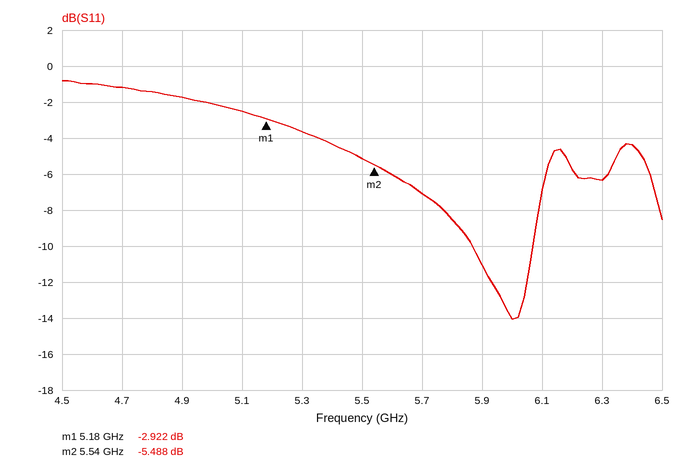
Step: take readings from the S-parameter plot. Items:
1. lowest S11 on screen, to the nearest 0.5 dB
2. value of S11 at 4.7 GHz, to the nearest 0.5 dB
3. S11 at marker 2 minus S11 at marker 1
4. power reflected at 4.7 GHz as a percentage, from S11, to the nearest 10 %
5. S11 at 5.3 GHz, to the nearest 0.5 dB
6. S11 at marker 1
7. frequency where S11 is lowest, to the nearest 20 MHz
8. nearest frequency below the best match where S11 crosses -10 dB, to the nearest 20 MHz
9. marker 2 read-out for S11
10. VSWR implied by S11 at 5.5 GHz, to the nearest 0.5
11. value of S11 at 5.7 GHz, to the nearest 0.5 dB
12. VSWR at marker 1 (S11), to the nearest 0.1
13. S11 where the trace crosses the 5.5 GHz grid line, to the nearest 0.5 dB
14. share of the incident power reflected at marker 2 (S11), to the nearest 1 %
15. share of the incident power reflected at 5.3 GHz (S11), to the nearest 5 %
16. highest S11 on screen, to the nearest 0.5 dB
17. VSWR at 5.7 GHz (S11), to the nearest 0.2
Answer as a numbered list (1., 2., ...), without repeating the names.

1. -14.0 dB
2. -1.0 dB
3. -2.566 dB
4. 80 %
5. -3.5 dB
6. -2.922 dB
7. 6.00 GHz
8. 5.86 GHz
9. -5.488 dB
10. 3.5
11. -7.0 dB
12. 6.0
13. -5.0 dB
14. 28 %
15. 45 %
16. -1.0 dB
17. 2.6
